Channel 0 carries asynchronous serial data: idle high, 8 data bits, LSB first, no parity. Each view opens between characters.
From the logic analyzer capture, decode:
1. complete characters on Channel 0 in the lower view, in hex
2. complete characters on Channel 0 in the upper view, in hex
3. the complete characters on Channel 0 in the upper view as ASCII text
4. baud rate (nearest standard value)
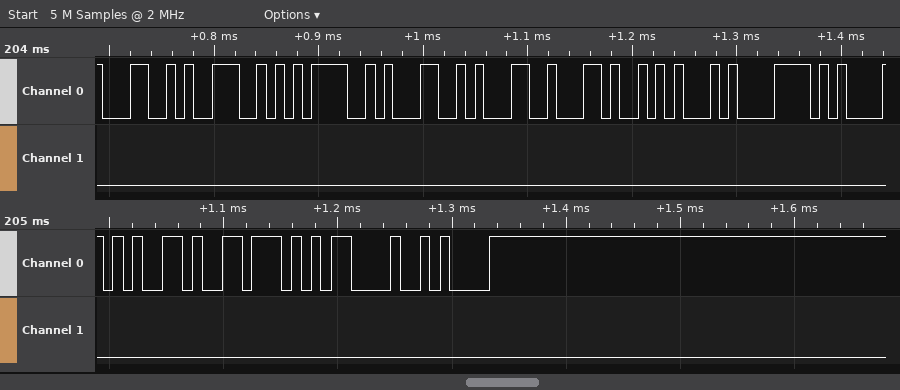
65, 76, 0D, 0A
4C, 4E, 3D, 31, 31, 2C, 45, 78
"LN=11,Ex"
115200 baud
